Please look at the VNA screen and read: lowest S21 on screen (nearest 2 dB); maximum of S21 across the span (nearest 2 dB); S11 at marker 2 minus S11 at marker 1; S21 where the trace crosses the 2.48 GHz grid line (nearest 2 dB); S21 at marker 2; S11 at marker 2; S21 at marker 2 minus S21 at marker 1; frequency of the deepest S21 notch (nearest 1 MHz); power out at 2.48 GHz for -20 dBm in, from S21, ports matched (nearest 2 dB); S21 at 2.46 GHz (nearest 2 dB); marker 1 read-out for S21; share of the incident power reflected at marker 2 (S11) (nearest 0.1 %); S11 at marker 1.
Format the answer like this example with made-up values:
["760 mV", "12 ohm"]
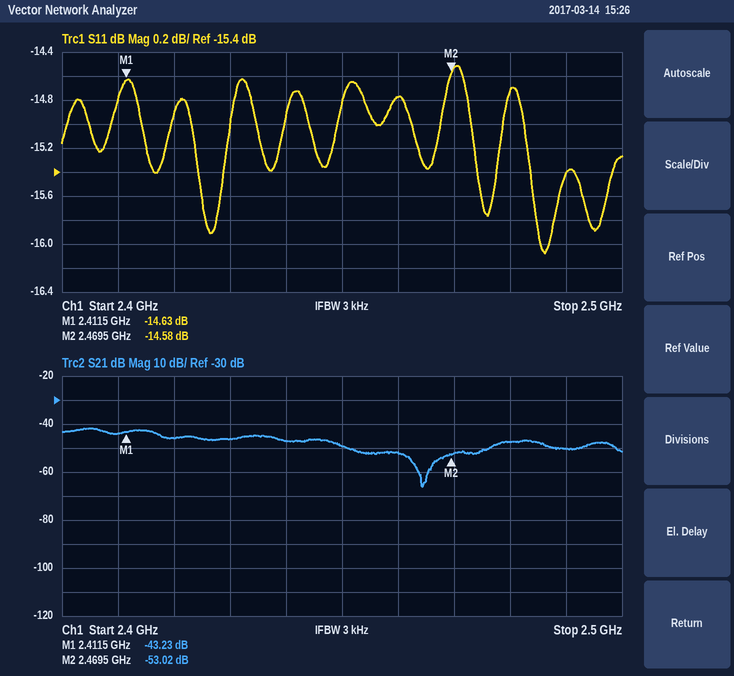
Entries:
["-66 dB", "-42 dB", "0.05 dB", "-48 dB", "-53.02 dB", "-14.58 dB", "-9.79 dB", "2.464 GHz", "-68 dBm", "-52 dB", "-43.23 dB", "3.5 %", "-14.63 dB"]
